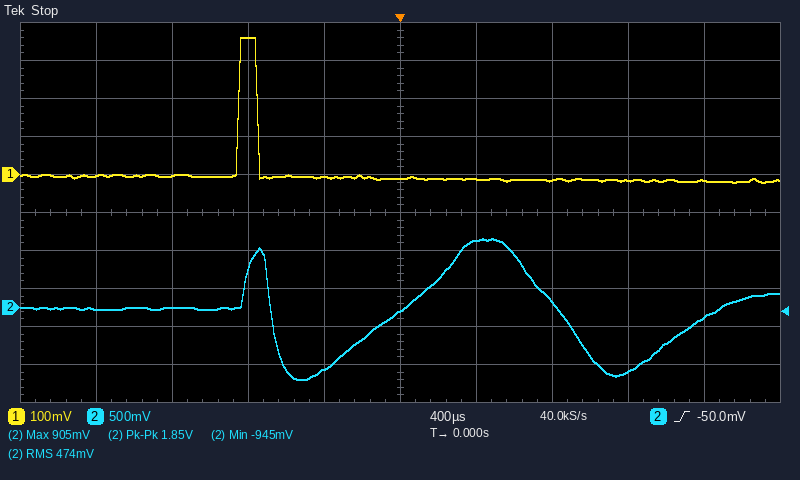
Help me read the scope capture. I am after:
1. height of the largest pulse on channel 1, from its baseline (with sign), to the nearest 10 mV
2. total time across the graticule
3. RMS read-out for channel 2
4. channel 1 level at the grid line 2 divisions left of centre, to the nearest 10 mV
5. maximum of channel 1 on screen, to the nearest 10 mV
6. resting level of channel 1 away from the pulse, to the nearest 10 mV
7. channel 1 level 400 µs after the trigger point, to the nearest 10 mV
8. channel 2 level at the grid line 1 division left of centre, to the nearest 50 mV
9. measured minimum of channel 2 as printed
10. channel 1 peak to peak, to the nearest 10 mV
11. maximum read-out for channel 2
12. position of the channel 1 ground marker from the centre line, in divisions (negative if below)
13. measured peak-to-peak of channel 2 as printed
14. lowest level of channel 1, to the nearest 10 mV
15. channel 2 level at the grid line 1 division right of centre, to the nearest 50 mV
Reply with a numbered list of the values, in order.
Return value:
1. +370 mV
2. 4 ms
3. 474 mV
4. 360 mV
5. 360 mV
6. -10 mV
7. -10 mV
8. -800 mV
9. -945 mV
10. 380 mV
11. 905 mV
12. +1.0 div
13. 1.85 V
14. -20 mV
15. 900 mV
